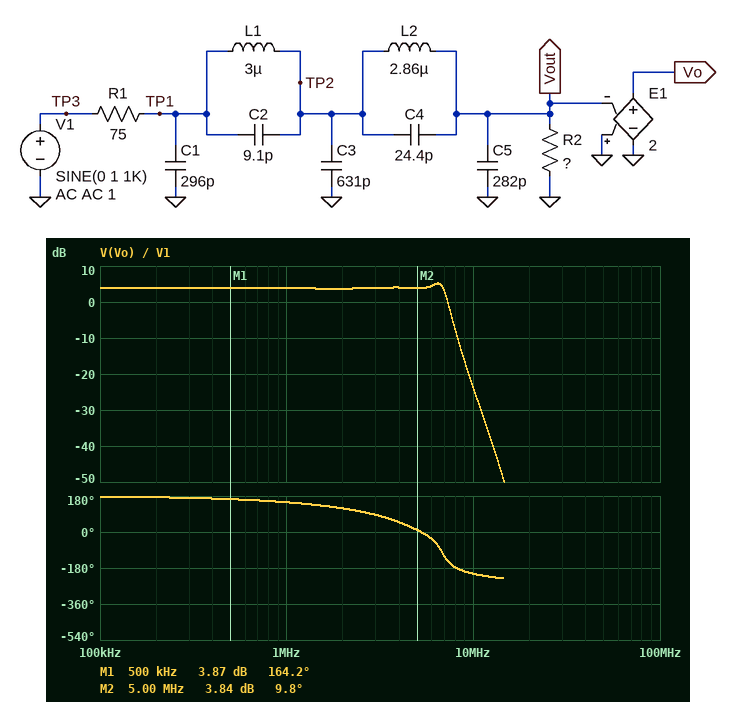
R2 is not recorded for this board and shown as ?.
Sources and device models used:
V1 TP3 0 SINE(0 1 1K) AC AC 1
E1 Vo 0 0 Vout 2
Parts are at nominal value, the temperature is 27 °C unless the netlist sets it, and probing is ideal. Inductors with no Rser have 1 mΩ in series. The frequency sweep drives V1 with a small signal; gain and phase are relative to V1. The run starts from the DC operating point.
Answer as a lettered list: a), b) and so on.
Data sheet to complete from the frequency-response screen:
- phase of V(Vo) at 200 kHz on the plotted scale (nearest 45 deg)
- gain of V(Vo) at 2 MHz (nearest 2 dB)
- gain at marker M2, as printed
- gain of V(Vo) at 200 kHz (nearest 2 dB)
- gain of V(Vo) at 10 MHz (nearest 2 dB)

a) 180 deg
b) 4 dB
c) 3.84 dB
d) 4 dB
e) -24 dB
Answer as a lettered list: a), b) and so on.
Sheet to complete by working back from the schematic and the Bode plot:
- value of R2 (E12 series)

a) 270 Ω
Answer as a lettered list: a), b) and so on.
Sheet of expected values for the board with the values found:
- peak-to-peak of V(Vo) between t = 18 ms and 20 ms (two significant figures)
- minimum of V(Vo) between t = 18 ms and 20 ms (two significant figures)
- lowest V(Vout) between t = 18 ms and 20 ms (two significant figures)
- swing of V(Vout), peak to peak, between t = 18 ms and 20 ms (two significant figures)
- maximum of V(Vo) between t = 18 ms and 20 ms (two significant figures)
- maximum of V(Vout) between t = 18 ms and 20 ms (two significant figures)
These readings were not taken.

a) 3.1 V
b) -1.6 V
c) -780 mV
d) 1.6 V
e) 1.6 V
f) 780 mV
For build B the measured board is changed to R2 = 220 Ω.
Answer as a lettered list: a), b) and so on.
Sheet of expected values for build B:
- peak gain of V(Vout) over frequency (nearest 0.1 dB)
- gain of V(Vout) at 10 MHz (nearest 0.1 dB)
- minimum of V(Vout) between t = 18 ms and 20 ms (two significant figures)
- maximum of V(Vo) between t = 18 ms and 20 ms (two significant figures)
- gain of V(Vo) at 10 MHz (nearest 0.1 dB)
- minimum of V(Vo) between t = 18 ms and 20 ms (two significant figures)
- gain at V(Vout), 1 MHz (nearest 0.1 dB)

a) -1.9 dB
b) -30.0 dB
c) -750 mV
d) 1.5 V
e) -24.0 dB
f) -1.5 V
g) -2.6 dB
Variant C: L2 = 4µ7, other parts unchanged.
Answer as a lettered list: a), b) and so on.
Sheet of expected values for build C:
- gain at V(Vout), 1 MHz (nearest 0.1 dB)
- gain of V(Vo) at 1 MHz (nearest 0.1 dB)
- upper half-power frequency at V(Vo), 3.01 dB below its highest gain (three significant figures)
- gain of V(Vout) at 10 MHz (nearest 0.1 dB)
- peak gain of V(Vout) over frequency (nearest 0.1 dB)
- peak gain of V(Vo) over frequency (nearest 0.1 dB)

a) -2.1 dB
b) 3.9 dB
c) 5.86 MHz
d) -38.7 dB
e) -0.5 dB
f) 5.5 dB
